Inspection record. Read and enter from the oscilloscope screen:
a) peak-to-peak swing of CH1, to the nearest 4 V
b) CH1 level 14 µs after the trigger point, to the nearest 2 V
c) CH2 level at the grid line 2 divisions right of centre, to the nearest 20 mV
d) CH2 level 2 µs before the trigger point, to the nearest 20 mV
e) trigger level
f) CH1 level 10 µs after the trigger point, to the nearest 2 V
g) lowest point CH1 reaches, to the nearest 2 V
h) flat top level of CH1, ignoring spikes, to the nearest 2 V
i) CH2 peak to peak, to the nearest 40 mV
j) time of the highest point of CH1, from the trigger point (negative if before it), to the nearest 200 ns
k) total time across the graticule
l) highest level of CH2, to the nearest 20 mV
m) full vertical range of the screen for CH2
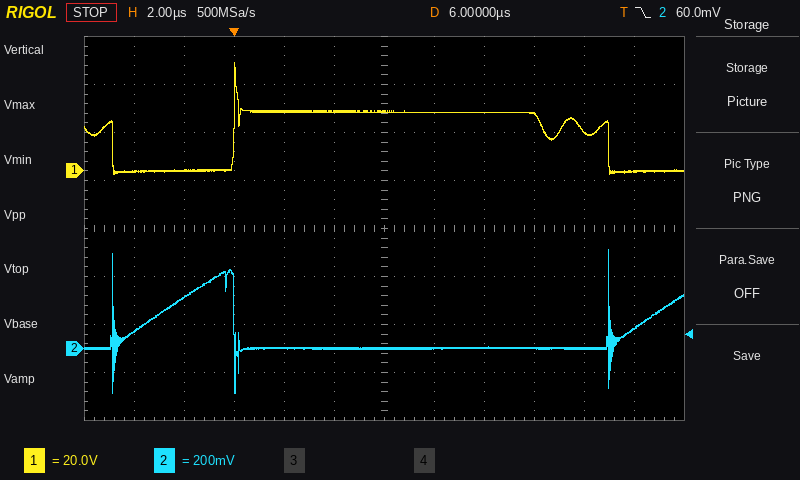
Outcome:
48 V
16 V
0 mV
220 mV
60.0 mV
24 V
-2 V
24 V
600 mV
0.0 µs
24 µs
420 mV
1.6 V
